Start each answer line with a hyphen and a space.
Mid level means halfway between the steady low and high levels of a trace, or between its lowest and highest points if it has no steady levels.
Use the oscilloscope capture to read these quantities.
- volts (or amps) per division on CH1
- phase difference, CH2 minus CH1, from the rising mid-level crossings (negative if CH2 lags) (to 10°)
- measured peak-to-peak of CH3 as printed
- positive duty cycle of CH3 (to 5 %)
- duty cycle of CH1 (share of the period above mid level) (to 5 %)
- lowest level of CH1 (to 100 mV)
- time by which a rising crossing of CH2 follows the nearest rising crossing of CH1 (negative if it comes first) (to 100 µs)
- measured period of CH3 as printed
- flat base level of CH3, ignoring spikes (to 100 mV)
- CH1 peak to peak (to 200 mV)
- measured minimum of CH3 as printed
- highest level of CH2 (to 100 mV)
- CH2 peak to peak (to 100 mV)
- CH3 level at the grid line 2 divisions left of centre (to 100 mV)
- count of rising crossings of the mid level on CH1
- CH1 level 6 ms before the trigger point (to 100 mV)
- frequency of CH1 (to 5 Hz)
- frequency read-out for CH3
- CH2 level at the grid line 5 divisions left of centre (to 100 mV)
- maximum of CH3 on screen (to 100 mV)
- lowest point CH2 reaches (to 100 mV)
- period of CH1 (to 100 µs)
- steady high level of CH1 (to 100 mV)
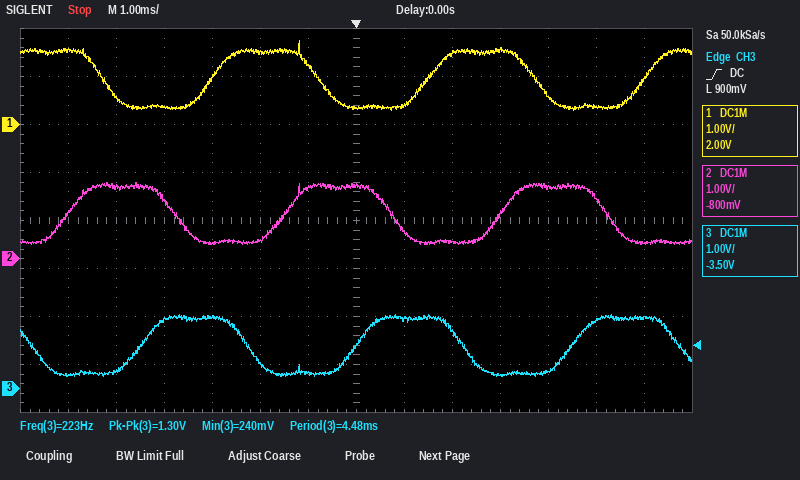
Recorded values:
- 1 V
- -120°
- 1.30 V
- 50 %
- 50 %
- 300 mV
- +1.5 ms
- 4.48 ms
- 300 mV
- 1.4 V
- 240 mV
- 1.6 V
- 1.3 V
- 500 mV
- 3
- 1.5 V
- 220 Hz
- 223 Hz
- 1.5 V
- 1.5 V
- 300 mV
- 4.5 ms
- 1.5 V
